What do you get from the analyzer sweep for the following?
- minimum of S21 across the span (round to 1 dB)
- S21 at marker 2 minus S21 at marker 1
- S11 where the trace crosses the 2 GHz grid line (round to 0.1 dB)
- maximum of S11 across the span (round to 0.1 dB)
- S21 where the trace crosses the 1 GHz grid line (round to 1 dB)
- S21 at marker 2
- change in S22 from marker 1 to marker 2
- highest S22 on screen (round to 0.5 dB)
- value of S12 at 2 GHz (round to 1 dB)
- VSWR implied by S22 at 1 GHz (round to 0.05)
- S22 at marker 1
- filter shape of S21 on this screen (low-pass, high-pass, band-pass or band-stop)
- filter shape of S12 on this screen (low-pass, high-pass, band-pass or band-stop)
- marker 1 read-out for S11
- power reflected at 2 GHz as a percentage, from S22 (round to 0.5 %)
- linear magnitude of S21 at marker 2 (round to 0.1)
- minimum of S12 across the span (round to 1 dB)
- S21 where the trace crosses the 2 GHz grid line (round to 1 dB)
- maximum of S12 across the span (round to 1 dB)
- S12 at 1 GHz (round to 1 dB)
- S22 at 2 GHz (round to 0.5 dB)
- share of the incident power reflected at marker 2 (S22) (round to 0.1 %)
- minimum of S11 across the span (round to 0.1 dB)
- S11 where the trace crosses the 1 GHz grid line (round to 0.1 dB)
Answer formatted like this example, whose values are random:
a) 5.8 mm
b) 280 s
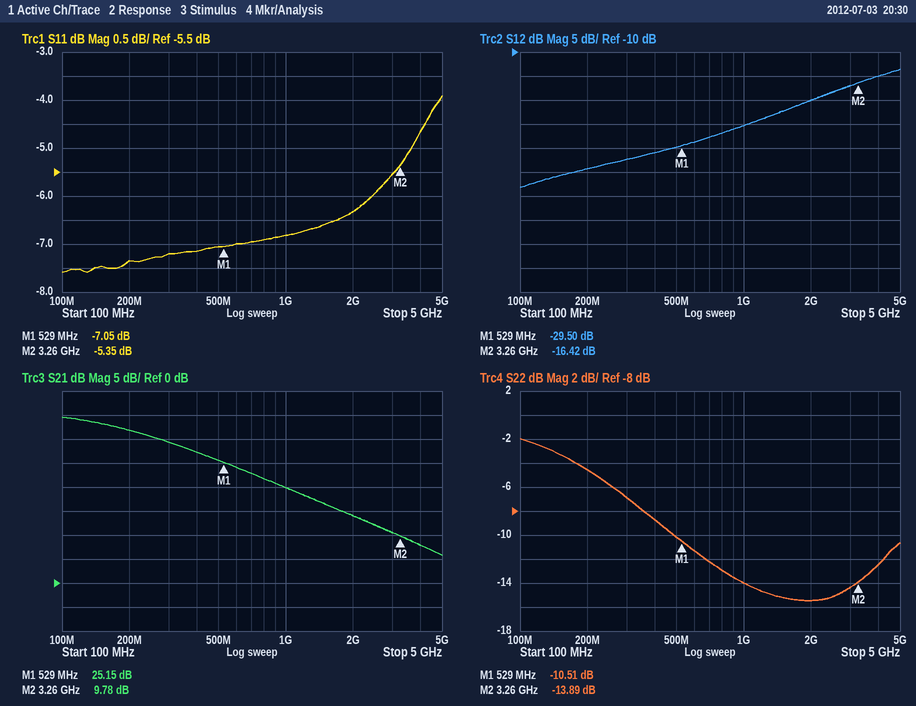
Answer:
a) 6 dB
b) -15.37 dB
c) -6.3 dB
d) -3.9 dB
e) 20 dB
f) 9.78 dB
g) -3.38 dB
h) -2.0 dB
i) -20 dB
j) 1.50
k) -10.51 dB
l) low-pass
m) high-pass
n) -7.05 dB
o) 3.0 %
p) 3.1
q) -38 dB
r) 14 dB
s) -14 dB
t) -25 dB
u) -15.5 dB
v) 4.1 %
w) -7.6 dB
x) -6.8 dB
